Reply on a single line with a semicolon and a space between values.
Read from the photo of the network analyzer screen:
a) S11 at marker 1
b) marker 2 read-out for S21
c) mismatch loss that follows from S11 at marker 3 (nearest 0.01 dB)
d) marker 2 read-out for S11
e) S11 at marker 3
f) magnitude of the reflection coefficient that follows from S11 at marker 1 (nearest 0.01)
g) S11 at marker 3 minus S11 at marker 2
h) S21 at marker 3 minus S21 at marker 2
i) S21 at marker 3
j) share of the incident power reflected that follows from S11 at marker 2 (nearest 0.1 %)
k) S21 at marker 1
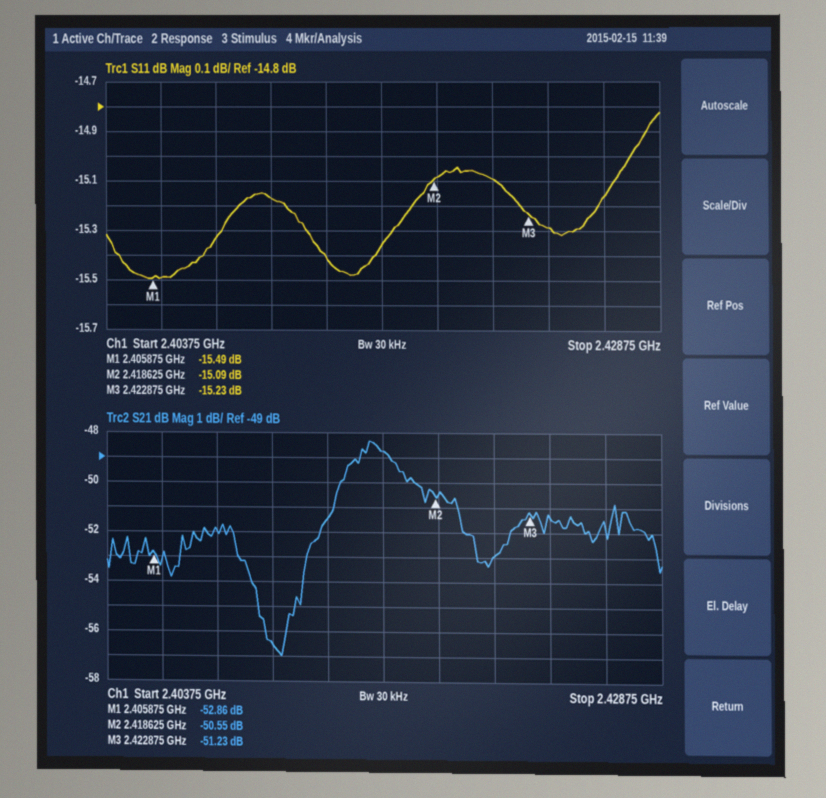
-15.49 dB; -50.55 dB; 0.13 dB; -15.09 dB; -15.23 dB; 0.17; -0.14 dB; -0.68 dB; -51.23 dB; 3.1 %; -52.86 dB
